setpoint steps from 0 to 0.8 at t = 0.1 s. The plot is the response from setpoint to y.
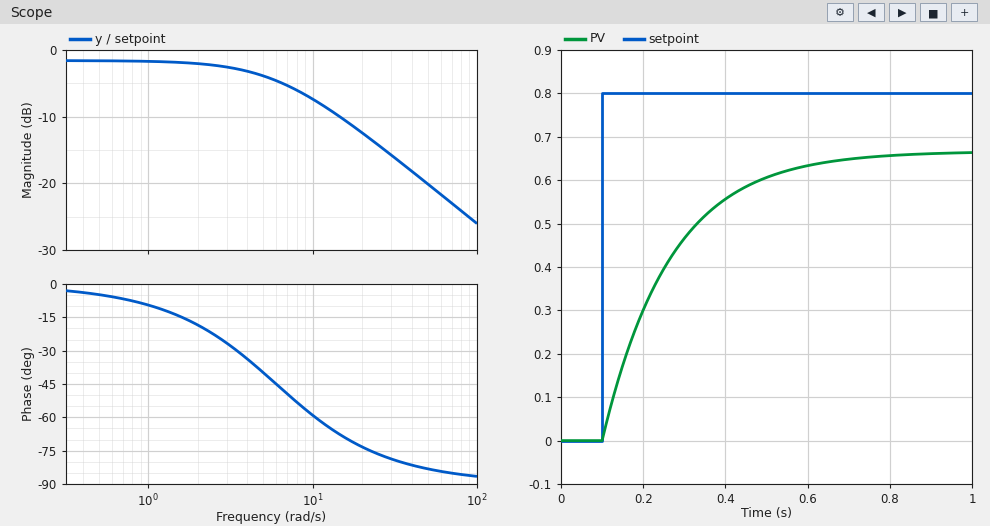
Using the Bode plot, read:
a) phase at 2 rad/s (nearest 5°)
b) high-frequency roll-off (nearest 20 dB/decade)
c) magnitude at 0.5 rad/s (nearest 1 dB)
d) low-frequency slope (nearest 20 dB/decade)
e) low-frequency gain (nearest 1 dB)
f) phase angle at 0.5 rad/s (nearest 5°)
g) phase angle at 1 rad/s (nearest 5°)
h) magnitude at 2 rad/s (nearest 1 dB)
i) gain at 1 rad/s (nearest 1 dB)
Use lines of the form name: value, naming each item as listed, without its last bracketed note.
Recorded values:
phase at 2 rad/s: -20°
high-frequency roll-off: -20 dB/decade
magnitude at 0.5 rad/s: -2 dB
low-frequency slope: 0 dB/decade
low-frequency gain: -2 dB
phase angle at 0.5 rad/s: -5°
phase angle at 1 rad/s: -10°
magnitude at 2 rad/s: -2 dB
gain at 1 rad/s: -2 dB
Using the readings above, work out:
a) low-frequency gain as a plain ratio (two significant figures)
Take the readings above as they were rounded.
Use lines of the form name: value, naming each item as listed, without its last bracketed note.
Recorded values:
low-frequency gain as a plain ratio: 0.79
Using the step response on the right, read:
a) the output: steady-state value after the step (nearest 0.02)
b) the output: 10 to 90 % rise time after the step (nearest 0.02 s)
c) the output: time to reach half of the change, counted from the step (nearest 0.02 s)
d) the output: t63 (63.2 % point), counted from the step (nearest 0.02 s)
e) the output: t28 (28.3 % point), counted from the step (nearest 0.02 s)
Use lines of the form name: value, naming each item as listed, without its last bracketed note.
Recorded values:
the output: steady-state value after the step: 0.66
the output: 10 to 90 % rise time after the step: 0.36 s
the output: time to reach half of the change, counted from the step: 0.12 s
the output: t63 (63.2 % point), counted from the step: 0.16 s
the output: t28 (28.3 % point), counted from the step: 0.06 s
